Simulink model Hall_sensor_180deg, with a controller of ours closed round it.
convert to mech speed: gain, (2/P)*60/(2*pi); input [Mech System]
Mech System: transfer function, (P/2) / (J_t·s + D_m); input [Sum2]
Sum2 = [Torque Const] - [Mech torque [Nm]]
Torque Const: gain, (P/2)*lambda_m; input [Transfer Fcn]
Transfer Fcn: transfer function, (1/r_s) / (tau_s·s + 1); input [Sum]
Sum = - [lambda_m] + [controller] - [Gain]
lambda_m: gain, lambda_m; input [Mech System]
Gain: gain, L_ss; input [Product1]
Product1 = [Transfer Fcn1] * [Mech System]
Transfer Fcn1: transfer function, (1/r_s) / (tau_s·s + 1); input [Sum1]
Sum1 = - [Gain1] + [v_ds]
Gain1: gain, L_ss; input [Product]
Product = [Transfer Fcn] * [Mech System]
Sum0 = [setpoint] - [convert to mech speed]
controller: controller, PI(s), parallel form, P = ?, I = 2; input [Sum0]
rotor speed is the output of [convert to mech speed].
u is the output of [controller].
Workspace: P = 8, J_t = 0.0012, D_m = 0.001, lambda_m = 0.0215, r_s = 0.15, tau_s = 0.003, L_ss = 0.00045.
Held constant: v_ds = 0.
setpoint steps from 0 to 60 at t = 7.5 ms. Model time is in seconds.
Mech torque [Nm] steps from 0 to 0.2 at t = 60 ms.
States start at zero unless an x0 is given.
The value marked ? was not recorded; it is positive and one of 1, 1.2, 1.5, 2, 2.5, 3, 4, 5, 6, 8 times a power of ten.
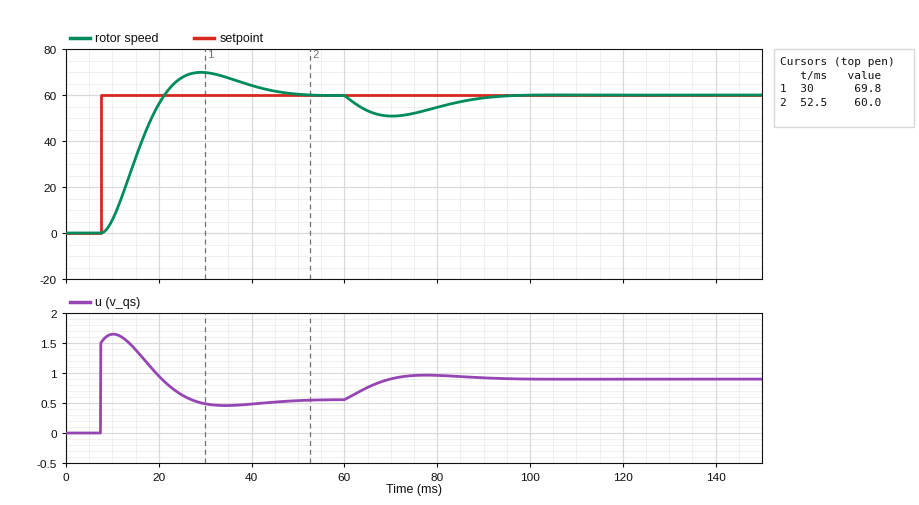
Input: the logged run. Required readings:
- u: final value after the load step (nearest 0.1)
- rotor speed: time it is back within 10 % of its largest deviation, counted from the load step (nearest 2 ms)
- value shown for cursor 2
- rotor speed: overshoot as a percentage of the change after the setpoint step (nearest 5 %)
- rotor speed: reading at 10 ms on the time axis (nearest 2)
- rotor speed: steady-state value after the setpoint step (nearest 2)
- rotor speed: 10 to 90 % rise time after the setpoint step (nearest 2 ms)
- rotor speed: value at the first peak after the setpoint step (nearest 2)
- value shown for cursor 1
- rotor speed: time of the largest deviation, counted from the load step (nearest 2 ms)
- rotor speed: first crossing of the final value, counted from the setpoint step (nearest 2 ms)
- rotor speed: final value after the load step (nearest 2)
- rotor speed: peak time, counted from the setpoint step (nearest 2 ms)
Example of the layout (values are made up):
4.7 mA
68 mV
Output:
0.9
32 ms
60.0
15 %
6
60
10 ms
70
69.8
10 ms
14 ms
60
22 ms
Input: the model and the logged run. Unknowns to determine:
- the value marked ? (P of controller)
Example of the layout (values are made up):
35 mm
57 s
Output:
0.025
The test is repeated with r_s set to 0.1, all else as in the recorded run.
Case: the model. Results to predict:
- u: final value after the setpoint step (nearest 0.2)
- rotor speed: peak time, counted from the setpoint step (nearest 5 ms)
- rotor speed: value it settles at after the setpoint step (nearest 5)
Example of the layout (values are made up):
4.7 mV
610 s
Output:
0.6
15 ms
60
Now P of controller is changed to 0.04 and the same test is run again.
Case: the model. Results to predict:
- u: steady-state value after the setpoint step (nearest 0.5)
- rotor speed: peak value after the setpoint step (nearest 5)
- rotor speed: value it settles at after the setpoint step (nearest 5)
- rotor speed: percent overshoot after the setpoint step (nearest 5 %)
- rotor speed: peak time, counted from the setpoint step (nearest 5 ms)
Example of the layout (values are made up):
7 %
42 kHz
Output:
0.5
65
60
10 %
15 ms
